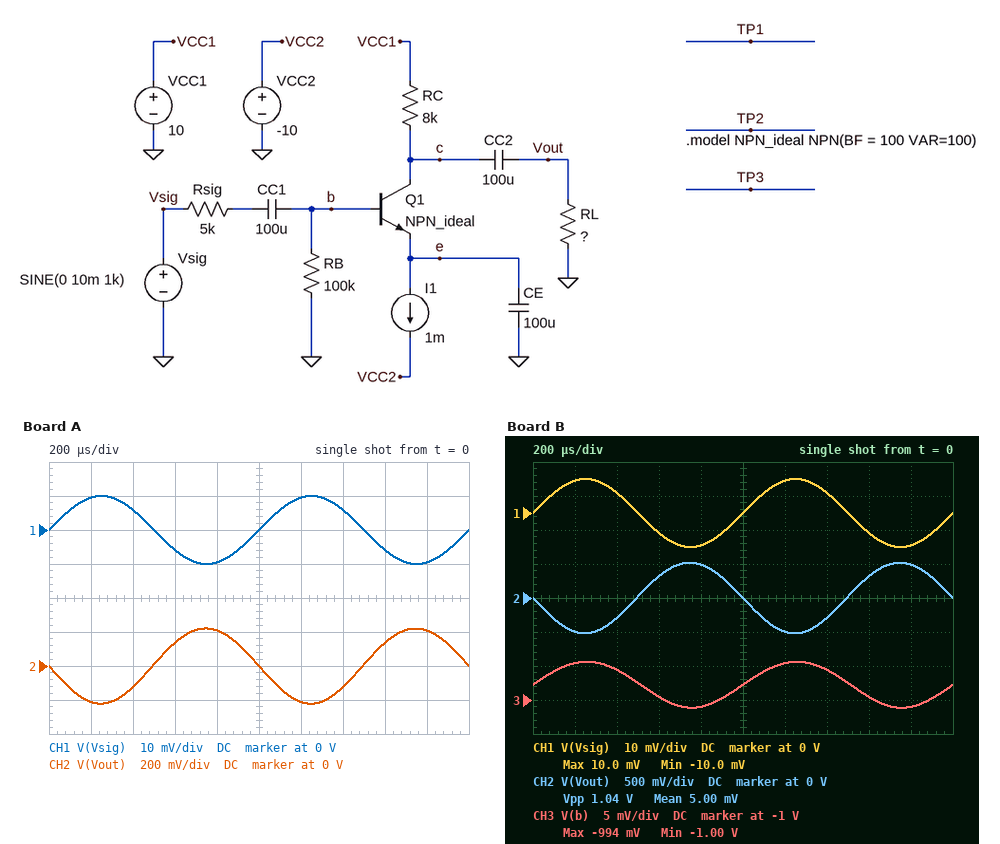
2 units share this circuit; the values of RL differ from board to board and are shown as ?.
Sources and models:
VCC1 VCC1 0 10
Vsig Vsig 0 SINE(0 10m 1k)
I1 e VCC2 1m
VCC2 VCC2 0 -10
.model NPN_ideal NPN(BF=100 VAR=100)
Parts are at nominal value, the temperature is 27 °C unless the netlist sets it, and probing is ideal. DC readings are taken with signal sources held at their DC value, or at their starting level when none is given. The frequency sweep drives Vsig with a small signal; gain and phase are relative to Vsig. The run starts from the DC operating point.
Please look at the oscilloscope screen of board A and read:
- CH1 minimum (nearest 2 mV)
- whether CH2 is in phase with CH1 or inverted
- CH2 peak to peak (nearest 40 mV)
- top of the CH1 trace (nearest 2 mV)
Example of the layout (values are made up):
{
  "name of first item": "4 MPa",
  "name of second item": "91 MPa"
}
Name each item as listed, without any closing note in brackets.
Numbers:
{
  "CH1 minimum": "-10 mV",
  "whether CH2 is in phase with CH1 or inverted": "inverted",
  "CH2 peak to peak": "440 mV",
  "top of the CH1 trace": "10 mV"
}
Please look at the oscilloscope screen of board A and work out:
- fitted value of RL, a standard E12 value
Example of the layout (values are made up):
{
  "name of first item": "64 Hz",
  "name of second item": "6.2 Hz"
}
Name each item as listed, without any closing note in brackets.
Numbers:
{
  "fitted value of RL, a standard E12 value": "2.2 kΩ"
}
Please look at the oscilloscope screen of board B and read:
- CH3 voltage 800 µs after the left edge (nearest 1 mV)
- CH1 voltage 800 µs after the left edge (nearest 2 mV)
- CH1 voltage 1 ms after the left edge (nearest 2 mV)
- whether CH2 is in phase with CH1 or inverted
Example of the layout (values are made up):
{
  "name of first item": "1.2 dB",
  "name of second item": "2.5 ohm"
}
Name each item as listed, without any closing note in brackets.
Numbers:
{
  "CH3 voltage 800 µs after the left edge": "-1.001 V",
  "CH1 voltage 800 µs after the left edge": "-10 mV",
  "CH1 voltage 1 ms after the left edge": "0 V",
  "whether CH2 is in phase with CH1 or inverted": "inverted"
}
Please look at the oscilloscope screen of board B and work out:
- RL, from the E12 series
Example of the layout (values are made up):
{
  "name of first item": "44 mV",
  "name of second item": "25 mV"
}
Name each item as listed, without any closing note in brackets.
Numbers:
{
  "RL, from the E12 series": "8.2 kΩ"
}
